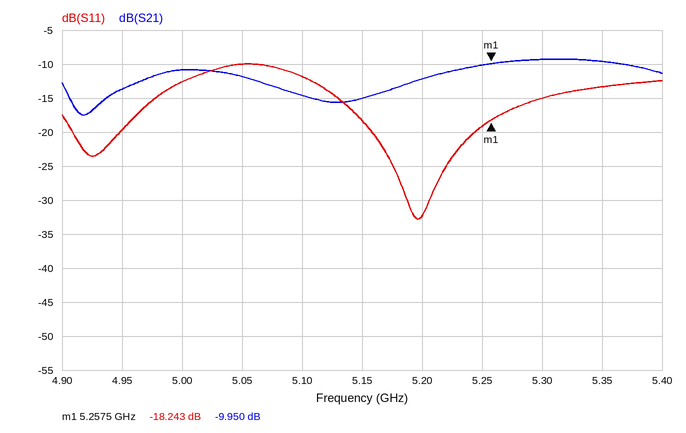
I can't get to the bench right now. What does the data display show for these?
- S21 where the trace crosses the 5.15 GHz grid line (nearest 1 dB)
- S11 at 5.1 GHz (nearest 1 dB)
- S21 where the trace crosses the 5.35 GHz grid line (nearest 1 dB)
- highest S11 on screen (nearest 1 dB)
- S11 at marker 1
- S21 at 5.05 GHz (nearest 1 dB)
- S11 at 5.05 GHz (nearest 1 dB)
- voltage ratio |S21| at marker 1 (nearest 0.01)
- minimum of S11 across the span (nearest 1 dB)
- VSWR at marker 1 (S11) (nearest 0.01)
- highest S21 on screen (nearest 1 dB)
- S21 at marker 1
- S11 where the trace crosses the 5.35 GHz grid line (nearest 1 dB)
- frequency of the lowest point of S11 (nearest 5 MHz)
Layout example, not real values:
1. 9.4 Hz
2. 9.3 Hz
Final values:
1. -15 dB
2. -12 dB
3. -10 dB
4. -10 dB
5. -18.243 dB
6. -12 dB
7. -10 dB
8. 0.32
9. -33 dB
10. 1.28
11. -9 dB
12. -9.950 dB
13. -13 dB
14. 5.195 GHz
